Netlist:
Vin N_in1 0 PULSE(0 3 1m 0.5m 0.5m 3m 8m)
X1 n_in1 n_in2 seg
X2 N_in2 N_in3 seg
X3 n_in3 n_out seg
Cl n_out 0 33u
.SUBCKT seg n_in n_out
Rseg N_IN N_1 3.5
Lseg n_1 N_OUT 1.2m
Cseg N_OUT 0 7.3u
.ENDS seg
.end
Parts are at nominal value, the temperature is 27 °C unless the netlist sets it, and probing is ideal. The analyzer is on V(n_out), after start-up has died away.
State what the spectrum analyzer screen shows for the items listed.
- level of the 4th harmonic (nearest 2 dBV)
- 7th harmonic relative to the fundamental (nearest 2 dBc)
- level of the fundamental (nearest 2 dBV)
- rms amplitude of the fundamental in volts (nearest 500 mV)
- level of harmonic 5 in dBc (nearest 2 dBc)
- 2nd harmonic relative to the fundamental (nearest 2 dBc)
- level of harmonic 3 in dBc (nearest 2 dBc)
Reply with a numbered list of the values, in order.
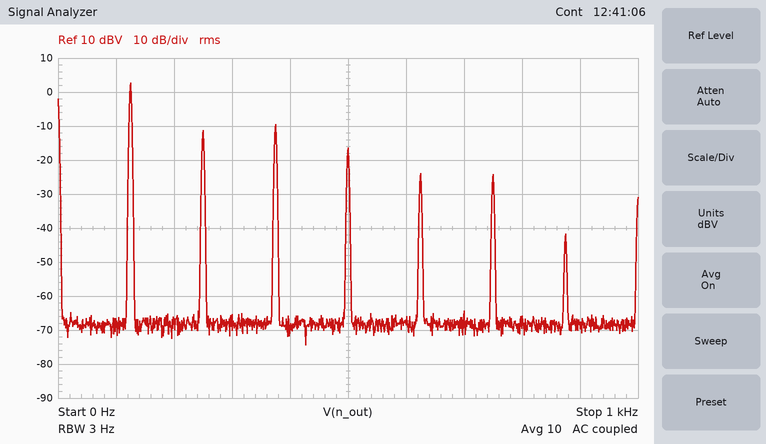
1. -16 dBV
2. -44 dBc
3. 2 dBV
4. 1.5 V
5. -26 dBc
6. -14 dBc
7. -12 dBc
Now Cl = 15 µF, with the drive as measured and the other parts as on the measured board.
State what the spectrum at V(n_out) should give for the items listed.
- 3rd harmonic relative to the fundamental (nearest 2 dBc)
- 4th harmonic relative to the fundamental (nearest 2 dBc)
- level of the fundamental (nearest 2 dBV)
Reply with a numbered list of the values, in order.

1. -10 dBc
2. -14 dBc
3. 2 dBV
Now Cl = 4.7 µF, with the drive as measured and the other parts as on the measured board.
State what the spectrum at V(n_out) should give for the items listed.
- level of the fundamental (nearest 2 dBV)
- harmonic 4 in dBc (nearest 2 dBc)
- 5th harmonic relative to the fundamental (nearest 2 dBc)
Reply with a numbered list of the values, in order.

1. 2 dBV
2. -12 dBc
3. -16 dBc
